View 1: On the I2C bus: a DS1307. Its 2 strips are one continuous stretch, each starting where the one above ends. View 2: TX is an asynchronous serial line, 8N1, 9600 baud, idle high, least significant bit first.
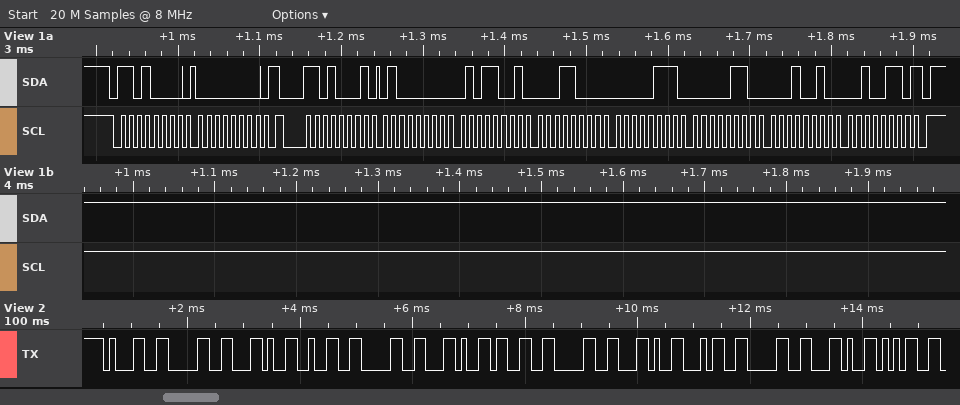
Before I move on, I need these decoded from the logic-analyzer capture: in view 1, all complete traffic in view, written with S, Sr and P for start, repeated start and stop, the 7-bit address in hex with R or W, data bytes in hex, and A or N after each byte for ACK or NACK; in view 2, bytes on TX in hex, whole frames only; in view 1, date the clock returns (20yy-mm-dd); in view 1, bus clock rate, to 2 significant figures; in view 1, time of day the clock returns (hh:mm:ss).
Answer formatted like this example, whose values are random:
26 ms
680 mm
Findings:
S 68W A 00 A Sr 68R A 40 A 59 A 18 A 07 A 06 A 12 A 26 N P
31 30 2C 32 30 2C 33 30 2C 34 30 2C 35
2026-12-06
100 kHz
18:59:40
